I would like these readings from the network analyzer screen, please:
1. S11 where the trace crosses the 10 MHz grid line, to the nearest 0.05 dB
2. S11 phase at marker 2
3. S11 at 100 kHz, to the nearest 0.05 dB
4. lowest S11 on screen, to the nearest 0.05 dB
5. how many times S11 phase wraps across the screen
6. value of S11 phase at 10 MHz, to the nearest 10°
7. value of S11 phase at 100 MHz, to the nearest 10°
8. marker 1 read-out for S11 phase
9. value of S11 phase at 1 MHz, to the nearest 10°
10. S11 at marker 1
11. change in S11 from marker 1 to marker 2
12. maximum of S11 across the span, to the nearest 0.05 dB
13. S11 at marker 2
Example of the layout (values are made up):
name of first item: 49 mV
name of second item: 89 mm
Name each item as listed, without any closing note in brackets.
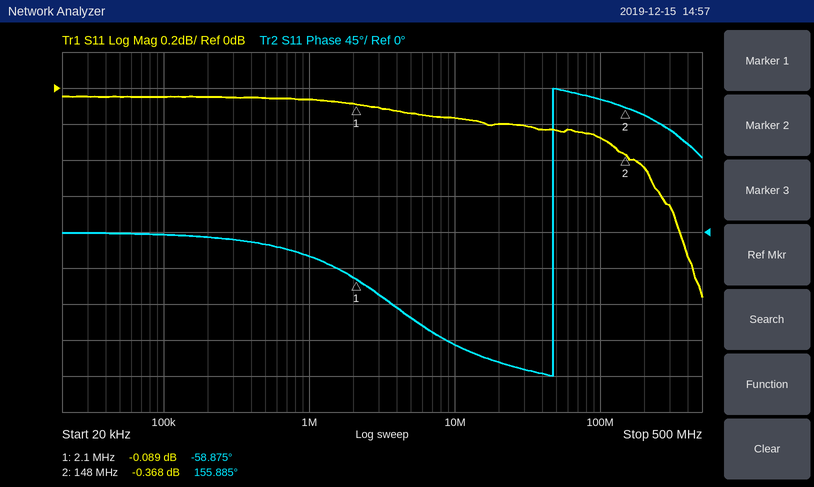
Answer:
S11 where the trace crosses the 10 MHz grid line, to the nearest 0.05 dB: -0.15 dB
S11 phase at marker 2: 155.885°
S11 at 100 kHz, to the nearest 0.05 dB: -0.05 dB
lowest S11 on screen, to the nearest 0.05 dB: -1.15 dB
how many times S11 phase wraps across the screen: 1
value of S11 phase at 10 MHz, to the nearest 10°: -140°
value of S11 phase at 100 MHz, to the nearest 10°: 170°
marker 1 read-out for S11 phase: -58.875°
value of S11 phase at 1 MHz, to the nearest 10°: -30°
S11 at marker 1: -0.089 dB
change in S11 from marker 1 to marker 2: -0.279 dB
maximum of S11 across the span, to the nearest 0.05 dB: -0.05 dB
S11 at marker 2: -0.368 dB
